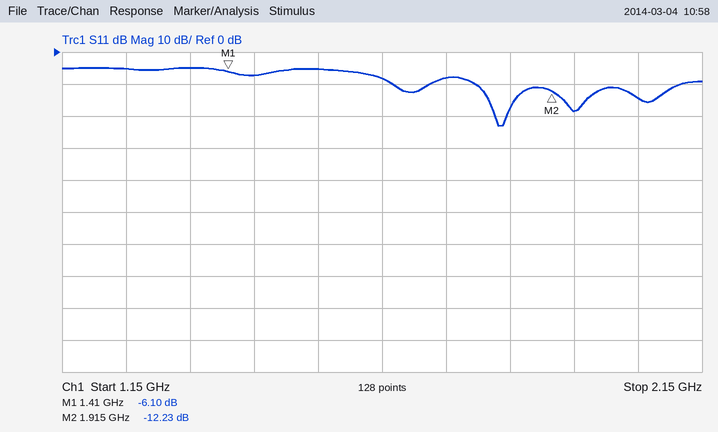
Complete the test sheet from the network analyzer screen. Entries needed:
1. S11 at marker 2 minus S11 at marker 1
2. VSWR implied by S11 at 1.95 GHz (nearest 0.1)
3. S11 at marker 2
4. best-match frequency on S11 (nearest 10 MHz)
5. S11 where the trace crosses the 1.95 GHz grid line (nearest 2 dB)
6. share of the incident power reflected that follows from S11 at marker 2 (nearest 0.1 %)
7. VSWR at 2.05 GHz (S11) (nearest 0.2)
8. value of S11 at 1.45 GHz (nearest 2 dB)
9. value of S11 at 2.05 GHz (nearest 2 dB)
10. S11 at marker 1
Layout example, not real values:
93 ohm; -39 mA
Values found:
-6.13 dB; 1.3; -12.23 dB; 1.83 GHz; -18 dB; 6.0 %; 1.4; -8 dB; -14 dB; -6.10 dB
